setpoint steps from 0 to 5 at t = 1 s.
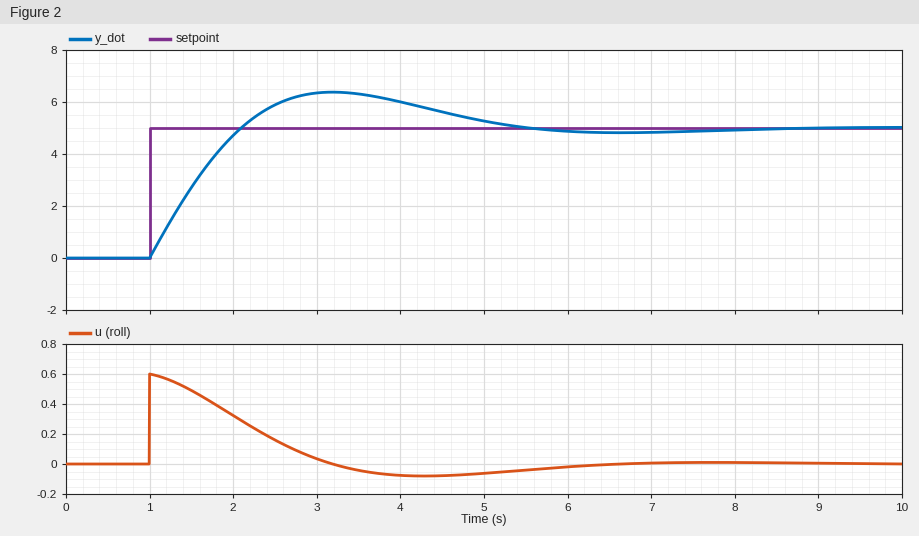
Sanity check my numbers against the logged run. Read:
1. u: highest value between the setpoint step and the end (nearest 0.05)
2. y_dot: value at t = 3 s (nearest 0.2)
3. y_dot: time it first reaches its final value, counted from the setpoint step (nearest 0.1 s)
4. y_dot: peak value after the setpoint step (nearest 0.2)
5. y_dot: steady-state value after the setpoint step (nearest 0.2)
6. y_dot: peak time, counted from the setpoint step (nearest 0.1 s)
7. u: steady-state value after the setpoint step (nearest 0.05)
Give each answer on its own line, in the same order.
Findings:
0.60
6.4
1.1 s
6.4
5.0
2.2 s
0.00
